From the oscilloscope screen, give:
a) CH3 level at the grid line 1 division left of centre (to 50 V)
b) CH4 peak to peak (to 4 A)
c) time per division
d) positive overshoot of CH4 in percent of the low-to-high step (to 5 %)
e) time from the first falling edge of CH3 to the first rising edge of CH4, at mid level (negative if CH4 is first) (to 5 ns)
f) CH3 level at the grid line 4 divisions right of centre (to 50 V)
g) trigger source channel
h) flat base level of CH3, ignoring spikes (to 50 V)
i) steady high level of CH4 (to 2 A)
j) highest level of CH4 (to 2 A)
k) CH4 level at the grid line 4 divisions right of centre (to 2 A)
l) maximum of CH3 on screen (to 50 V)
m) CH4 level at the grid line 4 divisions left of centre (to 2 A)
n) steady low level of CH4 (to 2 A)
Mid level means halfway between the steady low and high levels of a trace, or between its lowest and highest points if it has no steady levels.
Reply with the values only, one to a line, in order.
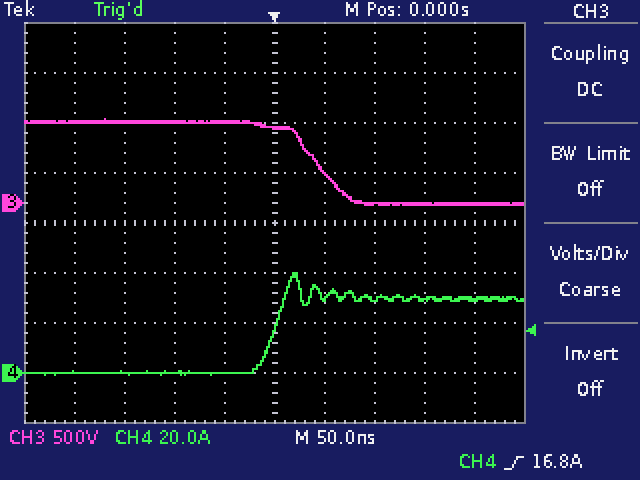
800 V
40 A
50 ns
35 %
-45 ns
0 V
CH4
0 V
30 A
40 A
30 A
850 V
0 A
0 A
